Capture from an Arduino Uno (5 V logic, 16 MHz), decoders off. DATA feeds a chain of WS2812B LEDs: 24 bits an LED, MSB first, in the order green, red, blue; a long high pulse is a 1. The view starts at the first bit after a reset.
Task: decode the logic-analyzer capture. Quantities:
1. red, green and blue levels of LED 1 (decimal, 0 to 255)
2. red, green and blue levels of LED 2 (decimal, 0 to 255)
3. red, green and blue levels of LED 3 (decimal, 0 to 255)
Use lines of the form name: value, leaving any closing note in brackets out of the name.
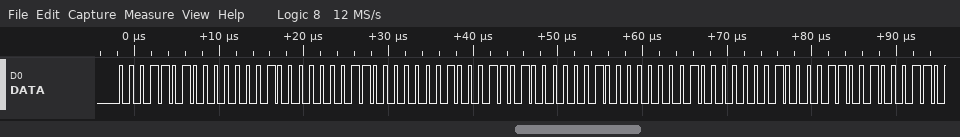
red, green and blue levels of LED 1: 2, 26, 3
red, green and blue levels of LED 2: 26, 1, 4
red, green and blue levels of LED 3: 2, 2, 25
